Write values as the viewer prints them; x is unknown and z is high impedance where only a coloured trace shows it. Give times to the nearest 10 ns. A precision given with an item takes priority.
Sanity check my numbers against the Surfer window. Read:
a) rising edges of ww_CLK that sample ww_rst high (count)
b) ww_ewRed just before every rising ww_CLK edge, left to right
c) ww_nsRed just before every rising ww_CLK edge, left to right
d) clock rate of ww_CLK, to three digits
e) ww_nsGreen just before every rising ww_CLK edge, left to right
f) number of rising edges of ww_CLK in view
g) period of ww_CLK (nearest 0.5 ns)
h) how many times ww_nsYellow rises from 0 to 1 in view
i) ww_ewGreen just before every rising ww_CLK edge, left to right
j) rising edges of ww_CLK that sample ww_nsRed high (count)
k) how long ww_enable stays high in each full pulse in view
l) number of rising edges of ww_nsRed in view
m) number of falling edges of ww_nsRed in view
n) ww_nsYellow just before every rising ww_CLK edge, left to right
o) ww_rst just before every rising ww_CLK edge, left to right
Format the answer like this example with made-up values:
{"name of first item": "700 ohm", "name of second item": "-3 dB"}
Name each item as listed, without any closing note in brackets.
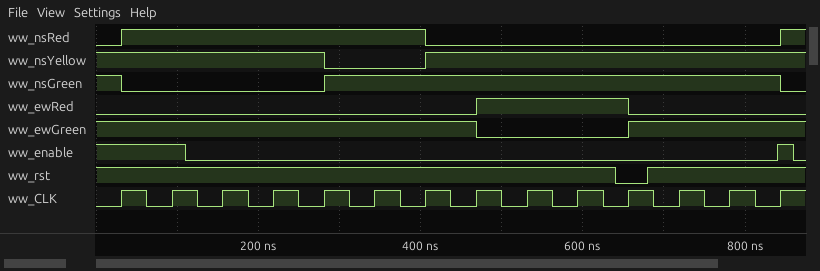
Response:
{"rising edges of ww_CLK that sample ww_rst high": "13", "ww_ewRed just before every rising ww_CLK edge, left to right": "0 0 0 0 0 0 0 0 1 1 1 0 0 0", "ww_nsRed just before every rising ww_CLK edge, left to right": "0 1 1 1 1 1 1 0 0 0 0 0 0 0", "clock rate of ww_CLK, to three digits": "16.0 MHz", "ww_nsGreen just before every rising ww_CLK edge, left to right": "1 0 0 0 0 1 1 1 1 1 1 1 1 1", "number of rising edges of ww_CLK in view": "14", "period of ww_CLK": "62.5 ns", "how many times ww_nsYellow rises from 0 to 1 in view": "1", "ww_ewGreen just before every rising ww_CLK edge, left to right": "1 1 1 1 1 1 1 1 0 0 0 1 1 1", "rising edges of ww_CLK that sample ww_nsRed high": "6", "how long ww_enable stays high in each full pulse in view": "20 ns", "number of rising edges of ww_nsRed in view": "2", "number of falling edges of ww_nsRed in view": "1", "ww_nsYellow just before every rising ww_CLK edge, left to right": "1 1 1 1 1 0 0 1 1 1 1 1 1 1", "ww_rst just before every rising ww_CLK edge, left to right": "1 1 1 1 1 1 1 1 1 1 0 1 1 1"}
